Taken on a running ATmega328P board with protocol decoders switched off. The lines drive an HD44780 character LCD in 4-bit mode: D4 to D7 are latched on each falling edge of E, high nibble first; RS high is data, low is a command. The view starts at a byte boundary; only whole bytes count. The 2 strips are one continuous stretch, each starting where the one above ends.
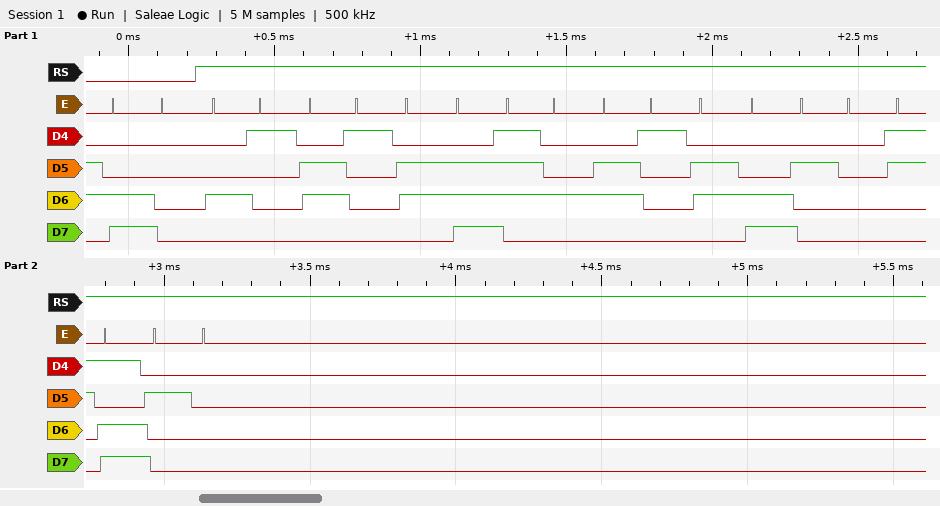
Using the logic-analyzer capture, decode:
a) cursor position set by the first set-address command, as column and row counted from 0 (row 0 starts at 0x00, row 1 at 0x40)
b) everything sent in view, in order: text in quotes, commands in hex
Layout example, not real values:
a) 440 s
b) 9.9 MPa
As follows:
a) column 0, row 1
b) 0xC0 "Aantal = "
